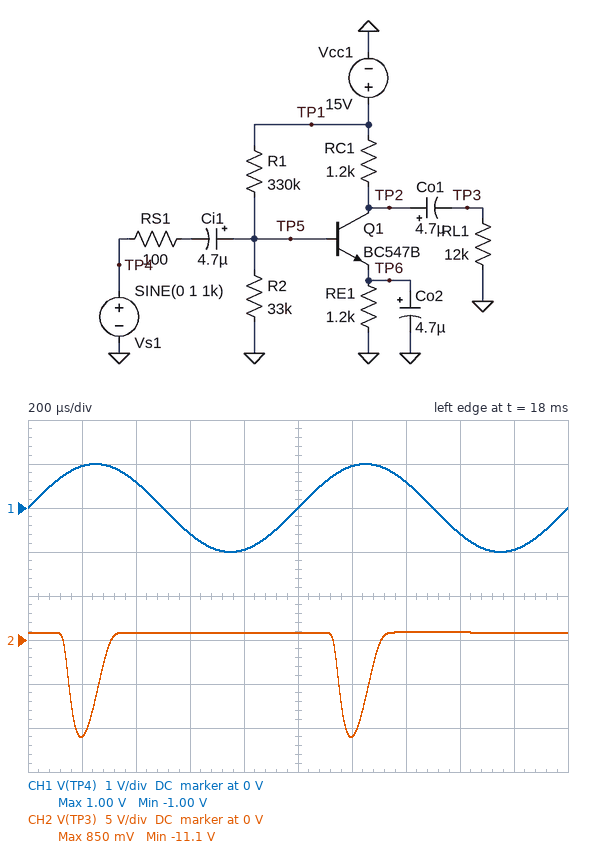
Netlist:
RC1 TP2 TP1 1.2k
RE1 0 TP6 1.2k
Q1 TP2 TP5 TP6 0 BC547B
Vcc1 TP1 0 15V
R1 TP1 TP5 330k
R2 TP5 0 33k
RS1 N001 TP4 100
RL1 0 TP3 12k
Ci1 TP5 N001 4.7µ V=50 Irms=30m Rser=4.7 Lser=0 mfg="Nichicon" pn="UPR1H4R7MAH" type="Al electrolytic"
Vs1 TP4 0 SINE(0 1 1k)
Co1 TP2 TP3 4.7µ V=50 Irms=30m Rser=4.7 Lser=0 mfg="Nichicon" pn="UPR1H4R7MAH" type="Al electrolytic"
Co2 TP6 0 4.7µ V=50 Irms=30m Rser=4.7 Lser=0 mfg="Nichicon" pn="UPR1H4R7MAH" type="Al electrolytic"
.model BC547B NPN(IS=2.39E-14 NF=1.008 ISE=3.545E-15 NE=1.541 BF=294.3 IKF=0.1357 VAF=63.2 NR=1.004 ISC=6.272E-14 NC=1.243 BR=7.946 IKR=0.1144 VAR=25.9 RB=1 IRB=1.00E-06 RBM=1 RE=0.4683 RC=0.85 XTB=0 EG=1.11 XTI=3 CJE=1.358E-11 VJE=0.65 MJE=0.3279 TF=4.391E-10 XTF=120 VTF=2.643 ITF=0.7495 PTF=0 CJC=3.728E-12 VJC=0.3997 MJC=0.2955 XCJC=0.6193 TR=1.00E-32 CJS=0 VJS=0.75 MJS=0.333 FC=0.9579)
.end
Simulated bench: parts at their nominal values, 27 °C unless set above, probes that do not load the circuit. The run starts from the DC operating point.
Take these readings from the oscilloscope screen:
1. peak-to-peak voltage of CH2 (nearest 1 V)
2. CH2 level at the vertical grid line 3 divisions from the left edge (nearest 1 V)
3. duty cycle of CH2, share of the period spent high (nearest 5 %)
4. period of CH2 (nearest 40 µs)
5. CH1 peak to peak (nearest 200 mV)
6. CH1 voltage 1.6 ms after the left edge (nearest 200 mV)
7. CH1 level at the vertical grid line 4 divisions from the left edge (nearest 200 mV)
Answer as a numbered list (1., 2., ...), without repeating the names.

1. 12 V
2. 1 V
3. 90 %
4. 1.00 ms
5. 2.0 V
6. -600 mV
7. -1.0 V
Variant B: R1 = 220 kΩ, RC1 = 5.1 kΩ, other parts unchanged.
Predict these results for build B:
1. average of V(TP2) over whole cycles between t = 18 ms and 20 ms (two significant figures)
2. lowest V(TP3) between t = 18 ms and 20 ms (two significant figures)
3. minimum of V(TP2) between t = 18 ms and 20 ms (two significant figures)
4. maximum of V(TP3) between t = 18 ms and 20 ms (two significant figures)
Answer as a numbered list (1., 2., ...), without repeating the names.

1. 11 V
2. -9.0 V
3. 1.1 V
4. 3.5 V
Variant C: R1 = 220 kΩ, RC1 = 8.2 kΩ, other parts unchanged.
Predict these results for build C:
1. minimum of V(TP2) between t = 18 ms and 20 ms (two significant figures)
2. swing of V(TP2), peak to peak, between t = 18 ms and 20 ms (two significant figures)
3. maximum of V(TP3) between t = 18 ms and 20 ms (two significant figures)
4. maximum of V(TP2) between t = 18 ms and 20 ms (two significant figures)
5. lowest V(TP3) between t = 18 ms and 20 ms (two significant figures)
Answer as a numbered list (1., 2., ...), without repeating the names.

1. 860 mV
2. 11 V
3. 4.6 V
4. 12 V
5. -6.5 V
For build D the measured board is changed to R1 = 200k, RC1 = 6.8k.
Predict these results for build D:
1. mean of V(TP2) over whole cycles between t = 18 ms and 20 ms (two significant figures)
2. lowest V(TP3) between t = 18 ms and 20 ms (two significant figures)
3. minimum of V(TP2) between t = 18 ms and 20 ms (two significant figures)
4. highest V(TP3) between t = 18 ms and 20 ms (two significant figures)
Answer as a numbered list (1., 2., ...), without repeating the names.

1. 10 V
2. -6.9 V
3. 970 mV
4. 4.6 V
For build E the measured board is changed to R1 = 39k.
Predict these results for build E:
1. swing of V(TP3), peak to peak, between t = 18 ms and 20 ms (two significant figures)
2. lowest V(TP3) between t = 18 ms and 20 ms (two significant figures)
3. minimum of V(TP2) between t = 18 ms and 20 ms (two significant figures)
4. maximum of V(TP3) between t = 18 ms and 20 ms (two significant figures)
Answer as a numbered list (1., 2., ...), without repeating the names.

1. 11 V
2. -5.8 V
3. 4.0 V
4. 4.8 V
